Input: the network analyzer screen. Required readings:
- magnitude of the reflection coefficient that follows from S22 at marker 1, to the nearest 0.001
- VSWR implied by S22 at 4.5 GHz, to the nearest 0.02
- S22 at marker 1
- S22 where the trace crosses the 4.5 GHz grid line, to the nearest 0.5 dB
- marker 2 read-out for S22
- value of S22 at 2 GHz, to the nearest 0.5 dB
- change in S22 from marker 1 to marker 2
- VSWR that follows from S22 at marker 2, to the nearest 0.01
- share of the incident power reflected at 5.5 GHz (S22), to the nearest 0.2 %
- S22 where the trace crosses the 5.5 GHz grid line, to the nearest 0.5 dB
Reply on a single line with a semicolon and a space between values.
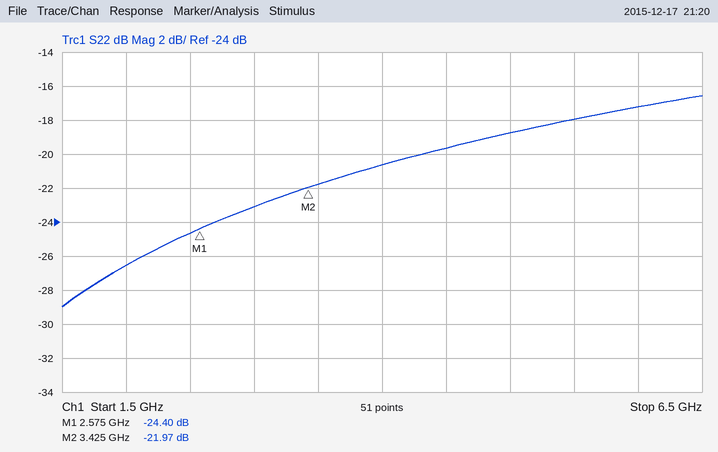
0.060; 1.24; -24.40 dB; -19.5 dB; -21.97 dB; -26.5 dB; 2.43 dB; 1.17; 1.6 %; -18.0 dB
